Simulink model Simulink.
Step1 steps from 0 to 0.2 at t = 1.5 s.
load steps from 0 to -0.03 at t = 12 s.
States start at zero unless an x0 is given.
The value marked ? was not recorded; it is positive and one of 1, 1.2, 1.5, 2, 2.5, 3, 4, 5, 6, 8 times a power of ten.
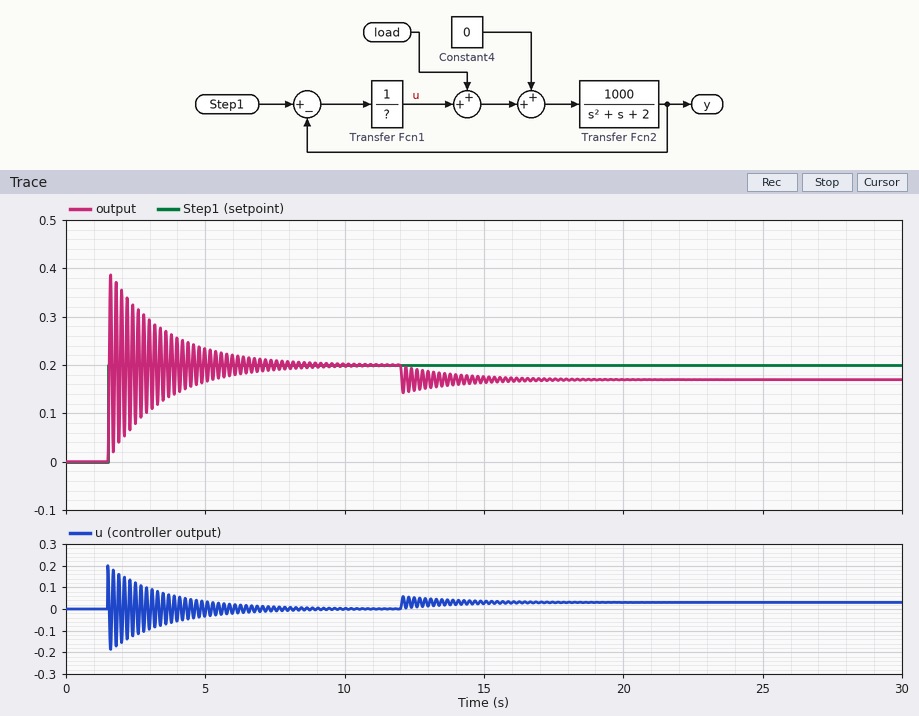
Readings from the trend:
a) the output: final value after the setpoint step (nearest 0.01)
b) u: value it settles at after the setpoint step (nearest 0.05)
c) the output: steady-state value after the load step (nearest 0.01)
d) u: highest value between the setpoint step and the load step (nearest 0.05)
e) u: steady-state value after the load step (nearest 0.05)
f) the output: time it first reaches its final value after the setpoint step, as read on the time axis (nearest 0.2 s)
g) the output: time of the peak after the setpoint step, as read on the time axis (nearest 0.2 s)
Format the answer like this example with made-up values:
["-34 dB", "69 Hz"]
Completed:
["0.20", "0.00", "0.17", "0.20", "0.05", "1.6 s", "1.6 s"]
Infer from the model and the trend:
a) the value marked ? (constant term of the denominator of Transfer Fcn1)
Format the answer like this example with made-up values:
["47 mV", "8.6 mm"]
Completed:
["1"]
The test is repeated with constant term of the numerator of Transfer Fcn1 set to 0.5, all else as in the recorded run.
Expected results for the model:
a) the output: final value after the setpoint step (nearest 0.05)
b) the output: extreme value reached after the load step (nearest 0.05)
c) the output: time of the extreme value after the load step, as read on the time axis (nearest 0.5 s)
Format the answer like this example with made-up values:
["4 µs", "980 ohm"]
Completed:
["0.20", "0.10", "12.0 s"]
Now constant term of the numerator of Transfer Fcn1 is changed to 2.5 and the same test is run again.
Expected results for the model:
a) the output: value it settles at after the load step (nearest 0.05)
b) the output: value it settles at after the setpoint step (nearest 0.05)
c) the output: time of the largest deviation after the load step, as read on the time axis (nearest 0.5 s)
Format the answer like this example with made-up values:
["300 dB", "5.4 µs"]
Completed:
["0.20", "0.20", "12.0 s"]
